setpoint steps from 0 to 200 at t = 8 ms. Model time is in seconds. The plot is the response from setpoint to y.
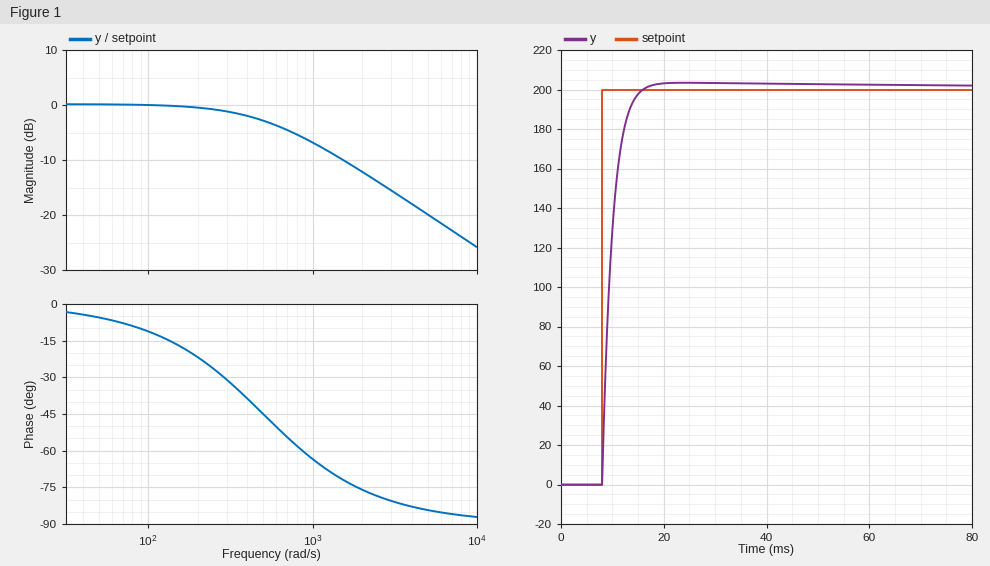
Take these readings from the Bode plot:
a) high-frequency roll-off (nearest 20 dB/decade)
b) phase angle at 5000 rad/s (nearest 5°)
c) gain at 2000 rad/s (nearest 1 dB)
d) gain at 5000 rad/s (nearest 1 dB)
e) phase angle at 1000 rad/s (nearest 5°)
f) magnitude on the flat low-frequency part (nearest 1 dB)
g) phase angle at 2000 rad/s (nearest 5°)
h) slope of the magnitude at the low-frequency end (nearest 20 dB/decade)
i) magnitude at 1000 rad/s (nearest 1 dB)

-20 dB/decade
-85°
-12 dB
-20 dB
-65°
0 dB
-75°
0 dB/decade
-7 dB
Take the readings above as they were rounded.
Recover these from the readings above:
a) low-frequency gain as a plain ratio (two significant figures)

1.0
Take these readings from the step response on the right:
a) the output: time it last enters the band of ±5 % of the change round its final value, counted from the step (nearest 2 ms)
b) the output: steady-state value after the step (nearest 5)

6 ms
200
